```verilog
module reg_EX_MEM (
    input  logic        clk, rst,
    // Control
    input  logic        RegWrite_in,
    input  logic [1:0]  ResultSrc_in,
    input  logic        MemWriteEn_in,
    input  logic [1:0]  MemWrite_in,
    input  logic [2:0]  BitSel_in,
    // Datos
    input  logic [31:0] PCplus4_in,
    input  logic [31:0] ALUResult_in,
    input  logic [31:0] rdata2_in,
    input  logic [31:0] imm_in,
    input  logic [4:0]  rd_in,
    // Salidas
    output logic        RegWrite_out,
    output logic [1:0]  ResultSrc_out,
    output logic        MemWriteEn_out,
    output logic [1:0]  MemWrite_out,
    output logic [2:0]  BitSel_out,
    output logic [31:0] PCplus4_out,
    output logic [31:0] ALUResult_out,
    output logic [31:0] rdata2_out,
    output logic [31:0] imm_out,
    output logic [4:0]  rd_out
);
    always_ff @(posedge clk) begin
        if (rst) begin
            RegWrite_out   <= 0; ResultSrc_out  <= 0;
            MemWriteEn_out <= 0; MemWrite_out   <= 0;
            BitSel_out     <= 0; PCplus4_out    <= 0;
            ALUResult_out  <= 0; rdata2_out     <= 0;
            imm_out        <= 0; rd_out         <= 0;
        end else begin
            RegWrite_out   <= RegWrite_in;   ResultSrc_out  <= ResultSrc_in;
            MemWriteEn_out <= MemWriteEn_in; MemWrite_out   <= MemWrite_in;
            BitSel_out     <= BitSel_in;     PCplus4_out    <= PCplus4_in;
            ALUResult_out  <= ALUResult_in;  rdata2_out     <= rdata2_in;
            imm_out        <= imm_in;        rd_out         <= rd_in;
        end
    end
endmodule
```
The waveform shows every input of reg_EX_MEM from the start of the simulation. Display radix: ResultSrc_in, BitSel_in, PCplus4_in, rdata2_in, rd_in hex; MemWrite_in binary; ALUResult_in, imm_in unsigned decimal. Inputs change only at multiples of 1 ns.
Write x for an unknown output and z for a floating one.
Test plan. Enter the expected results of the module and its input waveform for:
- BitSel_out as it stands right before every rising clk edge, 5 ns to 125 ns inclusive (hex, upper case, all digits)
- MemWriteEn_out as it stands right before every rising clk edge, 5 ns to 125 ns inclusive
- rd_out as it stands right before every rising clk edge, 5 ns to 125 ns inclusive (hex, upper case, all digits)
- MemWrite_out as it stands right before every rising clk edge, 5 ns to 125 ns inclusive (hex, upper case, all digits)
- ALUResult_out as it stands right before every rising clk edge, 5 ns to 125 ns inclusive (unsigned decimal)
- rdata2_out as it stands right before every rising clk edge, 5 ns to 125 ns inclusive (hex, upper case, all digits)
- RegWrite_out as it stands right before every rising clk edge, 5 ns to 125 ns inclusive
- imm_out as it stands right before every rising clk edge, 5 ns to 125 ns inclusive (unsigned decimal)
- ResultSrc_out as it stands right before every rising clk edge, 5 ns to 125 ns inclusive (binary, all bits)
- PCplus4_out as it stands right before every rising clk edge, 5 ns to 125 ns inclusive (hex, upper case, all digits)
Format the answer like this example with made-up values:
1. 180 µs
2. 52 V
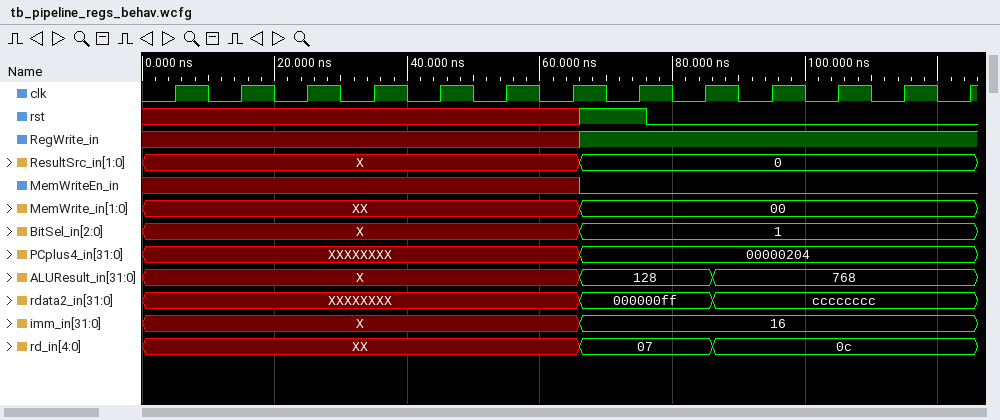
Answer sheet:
1. x, x, x, x, x, x, x, x, 0, 1, 1, 1, 1
2. x x x x x x x x 0 0 0 0 0
3. x, x, x, x, x, x, x, x, 00, 07, 0C, 0C, 0C
4. x, x, x, x, x, x, x, x, 0, 0, 0, 0, 0
5. x, x, x, x, x, x, x, x, 0, 128, 768, 768, 768
6. x, x, x, x, x, x, x, x, 00000000, 000000FF, CCCCCCCC, CCCCCCCC, CCCCCCCC
7. x x x x x x x x 0 1 1 1 1
8. x, x, x, x, x, x, x, x, 0, 16, 16, 16, 16
9. x, x, x, x, x, x, x, x, 00, 00, 00, 00, 00
10. x, x, x, x, x, x, x, x, 00000000, 00000204, 00000204, 00000204, 00000204
